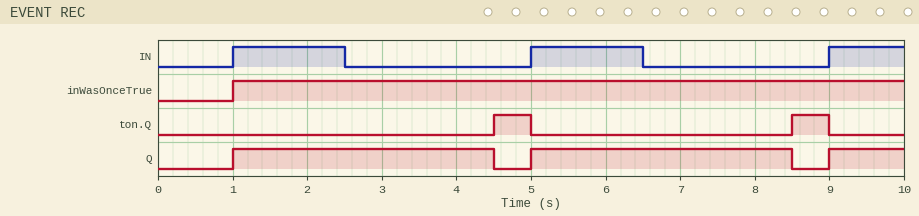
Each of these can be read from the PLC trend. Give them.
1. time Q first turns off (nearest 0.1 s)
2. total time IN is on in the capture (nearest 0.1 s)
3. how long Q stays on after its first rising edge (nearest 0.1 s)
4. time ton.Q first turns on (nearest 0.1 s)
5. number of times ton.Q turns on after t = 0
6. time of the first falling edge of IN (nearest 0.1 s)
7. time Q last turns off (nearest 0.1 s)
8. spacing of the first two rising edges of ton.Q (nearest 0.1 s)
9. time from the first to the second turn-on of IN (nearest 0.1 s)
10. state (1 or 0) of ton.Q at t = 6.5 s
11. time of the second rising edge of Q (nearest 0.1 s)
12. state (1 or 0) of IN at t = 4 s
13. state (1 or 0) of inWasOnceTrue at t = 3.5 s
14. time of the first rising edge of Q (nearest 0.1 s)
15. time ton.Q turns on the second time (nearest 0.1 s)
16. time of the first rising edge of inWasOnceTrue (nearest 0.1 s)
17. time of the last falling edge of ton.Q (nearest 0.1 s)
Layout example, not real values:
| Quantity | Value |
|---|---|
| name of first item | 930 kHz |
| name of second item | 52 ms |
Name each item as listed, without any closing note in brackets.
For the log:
| Quantity | Value |
|---|---|
| time Q first turns off | 4.5 s |
| total time IN is on in the capture | 4.0 s |
| how long Q stays on after its first rising edge | 3.5 s |
| time ton.Q first turns on | 4.5 s |
| number of times ton.Q turns on after t = 0 | 2 |
| time of the first falling edge of IN | 2.5 s |
| time Q last turns off | 8.5 s |
| spacing of the first two rising edges of ton.Q | 4.0 s |
| time from the first to the second turn-on of IN | 4.0 s |
| state (1 or 0) of ton.Q at t = 6.5 s | 0 |
| time of the second rising edge of Q | 5.0 s |
| state (1 or 0) of IN at t = 4 s | 0 |
| state (1 or 0) of inWasOnceTrue at t = 3.5 s | 1 |
| time of the first rising edge of Q | 1.0 s |
| time ton.Q turns on the second time | 8.5 s |
| time of the first rising edge of inWasOnceTrue | 1.0 s |
| time of the last falling edge of ton.Q | 9.0 s |
